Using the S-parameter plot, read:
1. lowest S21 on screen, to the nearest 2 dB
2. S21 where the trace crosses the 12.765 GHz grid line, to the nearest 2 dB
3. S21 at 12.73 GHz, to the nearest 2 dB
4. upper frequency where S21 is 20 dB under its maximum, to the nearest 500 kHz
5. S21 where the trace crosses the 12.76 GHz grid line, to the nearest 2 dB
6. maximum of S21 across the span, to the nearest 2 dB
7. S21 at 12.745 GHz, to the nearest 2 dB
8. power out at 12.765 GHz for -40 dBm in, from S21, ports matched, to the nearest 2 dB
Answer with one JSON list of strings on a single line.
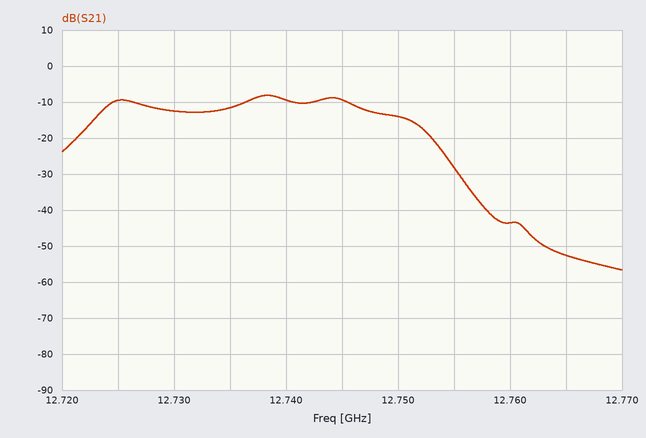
["-56 dB", "-52 dB", "-12 dB", "12.7550 GHz", "-44 dB", "-8 dB", "-10 dB", "-92 dBm"]
